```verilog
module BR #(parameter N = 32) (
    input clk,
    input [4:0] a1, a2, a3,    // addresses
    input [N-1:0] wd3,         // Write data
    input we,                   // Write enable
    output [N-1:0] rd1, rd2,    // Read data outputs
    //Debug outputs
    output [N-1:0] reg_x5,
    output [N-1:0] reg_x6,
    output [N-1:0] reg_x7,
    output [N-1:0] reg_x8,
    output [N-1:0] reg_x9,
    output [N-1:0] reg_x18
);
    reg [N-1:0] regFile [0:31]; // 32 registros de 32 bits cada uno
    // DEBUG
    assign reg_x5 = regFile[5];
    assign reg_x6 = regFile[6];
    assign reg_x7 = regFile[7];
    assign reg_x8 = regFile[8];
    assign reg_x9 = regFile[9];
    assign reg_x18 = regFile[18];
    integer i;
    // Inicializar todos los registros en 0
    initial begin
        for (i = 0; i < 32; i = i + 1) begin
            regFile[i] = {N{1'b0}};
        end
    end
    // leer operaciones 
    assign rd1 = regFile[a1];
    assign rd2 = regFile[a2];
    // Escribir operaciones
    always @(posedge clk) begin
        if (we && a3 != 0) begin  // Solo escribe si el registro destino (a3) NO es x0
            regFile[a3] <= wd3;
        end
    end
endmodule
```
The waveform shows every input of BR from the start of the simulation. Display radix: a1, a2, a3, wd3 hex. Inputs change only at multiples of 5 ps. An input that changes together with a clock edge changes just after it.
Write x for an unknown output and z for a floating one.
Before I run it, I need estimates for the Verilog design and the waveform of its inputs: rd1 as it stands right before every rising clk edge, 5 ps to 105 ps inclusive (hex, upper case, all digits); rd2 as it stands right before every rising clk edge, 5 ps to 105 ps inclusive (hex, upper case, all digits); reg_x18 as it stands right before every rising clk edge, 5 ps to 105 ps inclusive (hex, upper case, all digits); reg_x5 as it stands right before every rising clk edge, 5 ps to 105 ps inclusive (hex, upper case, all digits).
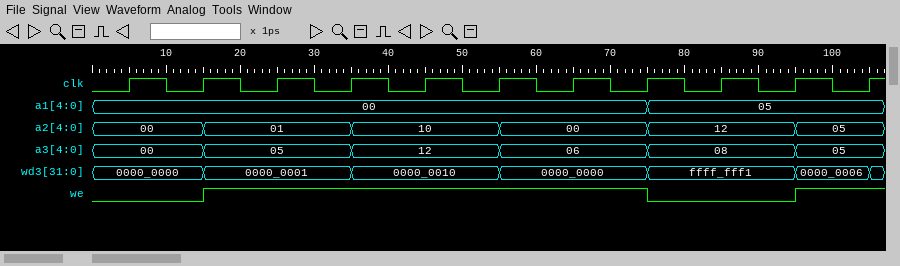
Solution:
00000000, 00000000, 00000000, 00000000, 00000000, 00000000, 00000000, 00000000, 00000001, 00000001, 00000001
00000000, 00000000, 00000000, 00000000, 00000000, 00000000, 00000000, 00000000, 00000010, 00000010, 00000001
00000000, 00000000, 00000000, 00000000, 00000000, 00000010, 00000010, 00000010, 00000010, 00000010, 00000010
00000000, 00000000, 00000000, 00000001, 00000001, 00000001, 00000001, 00000001, 00000001, 00000001, 00000001
